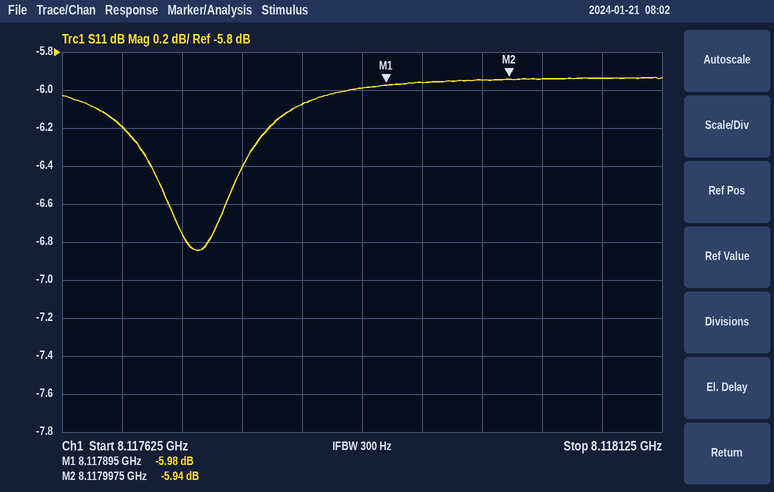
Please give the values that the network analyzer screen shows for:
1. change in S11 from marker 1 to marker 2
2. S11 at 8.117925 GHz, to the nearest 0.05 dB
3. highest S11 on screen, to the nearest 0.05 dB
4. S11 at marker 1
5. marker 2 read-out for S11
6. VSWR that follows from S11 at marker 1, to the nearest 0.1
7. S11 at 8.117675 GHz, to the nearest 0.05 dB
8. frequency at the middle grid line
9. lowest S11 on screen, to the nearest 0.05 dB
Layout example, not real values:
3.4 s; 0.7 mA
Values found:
0.04 dB; -5.95 dB; -5.95 dB; -5.98 dB; -5.94 dB; 3.0; -6.20 dB; 8.117875 GHz; -6.85 dB
